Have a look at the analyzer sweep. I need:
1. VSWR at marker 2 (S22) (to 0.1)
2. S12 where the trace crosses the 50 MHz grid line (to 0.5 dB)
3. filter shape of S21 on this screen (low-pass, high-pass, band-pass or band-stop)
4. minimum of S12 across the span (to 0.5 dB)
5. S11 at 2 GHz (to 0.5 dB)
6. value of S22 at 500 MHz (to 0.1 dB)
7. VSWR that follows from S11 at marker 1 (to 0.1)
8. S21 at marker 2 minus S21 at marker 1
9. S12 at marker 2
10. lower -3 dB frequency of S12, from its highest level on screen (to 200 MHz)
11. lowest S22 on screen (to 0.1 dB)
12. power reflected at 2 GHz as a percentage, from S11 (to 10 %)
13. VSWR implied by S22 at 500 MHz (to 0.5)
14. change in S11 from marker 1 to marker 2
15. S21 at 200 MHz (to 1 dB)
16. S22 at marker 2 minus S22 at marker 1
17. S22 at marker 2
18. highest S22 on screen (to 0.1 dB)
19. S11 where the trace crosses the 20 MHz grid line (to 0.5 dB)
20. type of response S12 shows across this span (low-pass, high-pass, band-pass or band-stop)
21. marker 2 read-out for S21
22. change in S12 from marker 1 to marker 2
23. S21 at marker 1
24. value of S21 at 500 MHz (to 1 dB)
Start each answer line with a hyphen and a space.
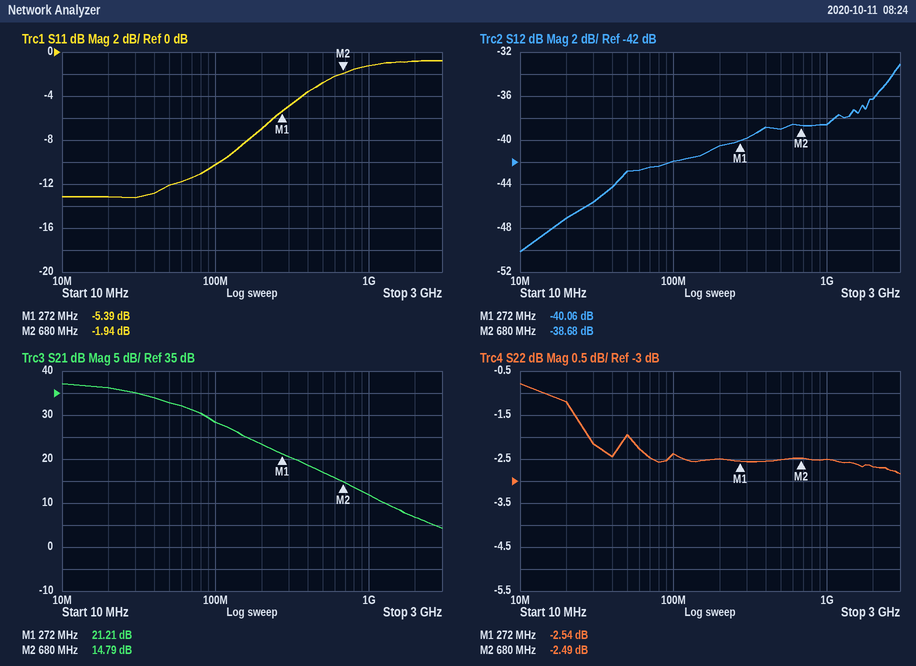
- 7.0
- -43.0 dB
- low-pass
- -50.0 dB
- -1.0 dB
- -2.5 dB
- 3.3
- -6.42 dB
- -38.68 dB
- 2.0 GHz
- -2.8 dB
- 80 %
- 7.0
- 3.45 dB
- 23 dB
- 0.05 dB
- -2.49 dB
- -0.8 dB
- -13.0 dB
- high-pass
- 14.79 dB
- 1.38 dB
- 21.21 dB
- 17 dB
